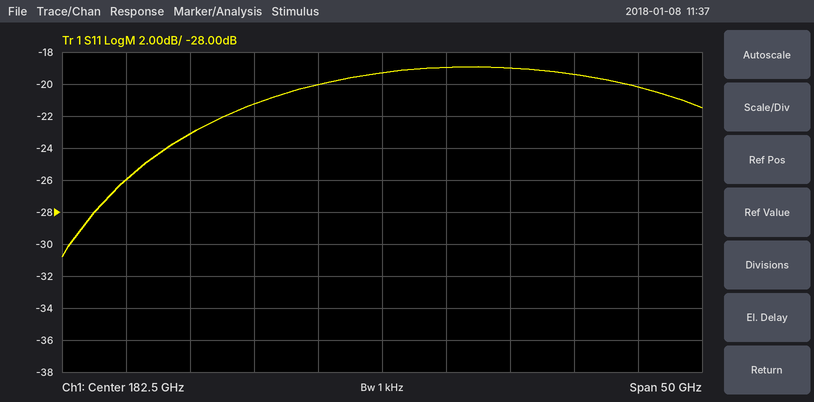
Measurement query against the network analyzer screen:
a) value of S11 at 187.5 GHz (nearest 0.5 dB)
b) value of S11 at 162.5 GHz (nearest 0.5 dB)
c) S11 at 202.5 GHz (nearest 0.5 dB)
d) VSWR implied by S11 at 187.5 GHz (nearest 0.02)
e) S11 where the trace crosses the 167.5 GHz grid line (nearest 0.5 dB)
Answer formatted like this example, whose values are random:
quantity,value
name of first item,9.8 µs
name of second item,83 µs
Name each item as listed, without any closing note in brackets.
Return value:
quantity,value
value of S11 at 187.5 GHz,-19.0 dB
value of S11 at 162.5 GHz,-26.0 dB
S11 at 202.5 GHz,-20.0 dB
VSWR implied by S11 at 187.5 GHz,1.26
S11 where the trace crosses the 167.5 GHz grid line,-23.0 dB
